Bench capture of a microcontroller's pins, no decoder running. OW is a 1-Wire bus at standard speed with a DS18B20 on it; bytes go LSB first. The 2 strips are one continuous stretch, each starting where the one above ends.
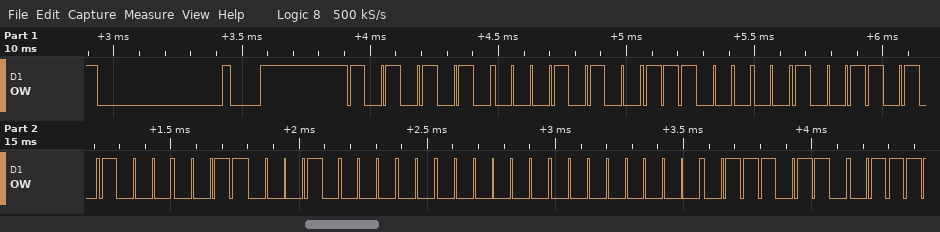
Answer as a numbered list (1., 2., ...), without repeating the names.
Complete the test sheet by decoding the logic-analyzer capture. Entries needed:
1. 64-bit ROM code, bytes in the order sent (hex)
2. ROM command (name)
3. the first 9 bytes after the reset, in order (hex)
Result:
1. 28 07 59 C1 08 00 00 6E
2. Match ROM
3. 55 28 07 59 C1 08 00 00 6E
